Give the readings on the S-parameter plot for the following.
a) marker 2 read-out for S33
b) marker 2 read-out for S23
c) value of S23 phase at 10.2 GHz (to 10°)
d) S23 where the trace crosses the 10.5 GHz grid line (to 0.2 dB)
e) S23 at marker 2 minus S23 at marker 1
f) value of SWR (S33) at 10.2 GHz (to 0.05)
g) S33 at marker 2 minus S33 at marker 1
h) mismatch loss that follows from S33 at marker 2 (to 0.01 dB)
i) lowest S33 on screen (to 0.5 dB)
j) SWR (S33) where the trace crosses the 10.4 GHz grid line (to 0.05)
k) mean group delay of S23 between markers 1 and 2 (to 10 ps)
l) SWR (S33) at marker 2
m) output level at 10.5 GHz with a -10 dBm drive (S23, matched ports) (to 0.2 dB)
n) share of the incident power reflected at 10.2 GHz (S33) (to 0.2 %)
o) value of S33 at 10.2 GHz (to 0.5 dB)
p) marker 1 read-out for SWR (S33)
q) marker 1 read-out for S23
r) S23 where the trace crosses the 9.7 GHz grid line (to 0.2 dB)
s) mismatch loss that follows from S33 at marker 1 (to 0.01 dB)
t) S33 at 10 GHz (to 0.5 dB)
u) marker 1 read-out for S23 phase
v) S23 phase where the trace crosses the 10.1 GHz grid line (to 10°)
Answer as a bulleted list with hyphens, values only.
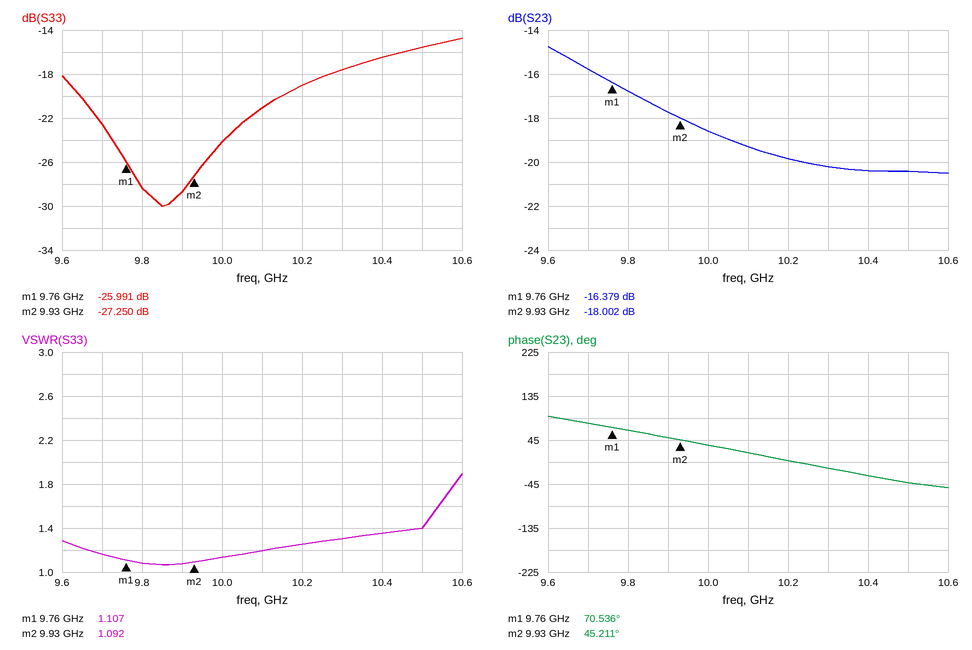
- -27.250 dB
- -18.002 dB
- 0°
- -20.4 dB
- -1.623 dB
- 1.25
- -1.259 dB
- 0.01 dB
- -30.0 dB
- 1.35
- 410 ps
- 1.092
- -30.4 dBm
- 1.2 %
- -19.0 dB
- 1.107
- -16.379 dB
- -15.8 dB
- 0.01 dB
- -24.0 dB
- 70.536°
- 20°
